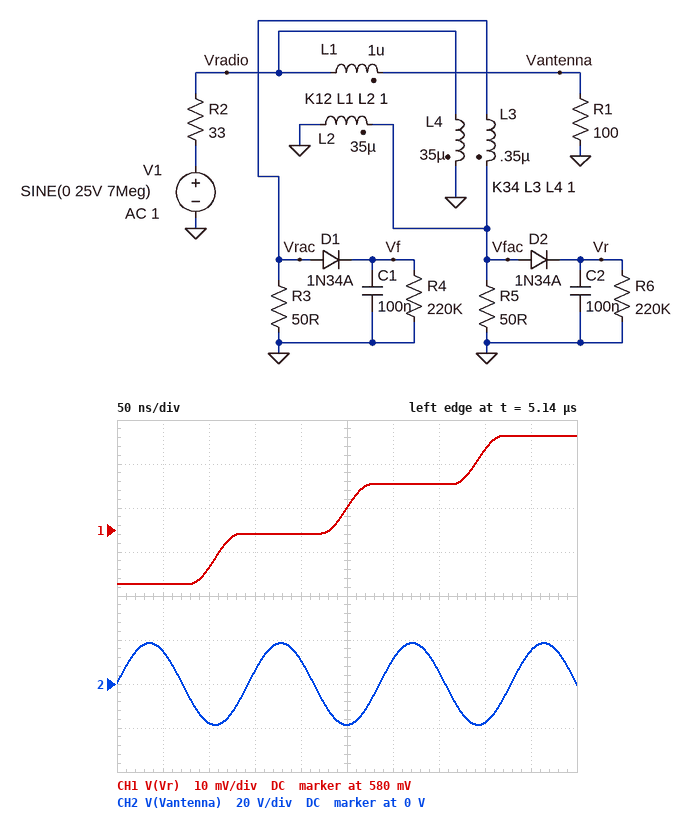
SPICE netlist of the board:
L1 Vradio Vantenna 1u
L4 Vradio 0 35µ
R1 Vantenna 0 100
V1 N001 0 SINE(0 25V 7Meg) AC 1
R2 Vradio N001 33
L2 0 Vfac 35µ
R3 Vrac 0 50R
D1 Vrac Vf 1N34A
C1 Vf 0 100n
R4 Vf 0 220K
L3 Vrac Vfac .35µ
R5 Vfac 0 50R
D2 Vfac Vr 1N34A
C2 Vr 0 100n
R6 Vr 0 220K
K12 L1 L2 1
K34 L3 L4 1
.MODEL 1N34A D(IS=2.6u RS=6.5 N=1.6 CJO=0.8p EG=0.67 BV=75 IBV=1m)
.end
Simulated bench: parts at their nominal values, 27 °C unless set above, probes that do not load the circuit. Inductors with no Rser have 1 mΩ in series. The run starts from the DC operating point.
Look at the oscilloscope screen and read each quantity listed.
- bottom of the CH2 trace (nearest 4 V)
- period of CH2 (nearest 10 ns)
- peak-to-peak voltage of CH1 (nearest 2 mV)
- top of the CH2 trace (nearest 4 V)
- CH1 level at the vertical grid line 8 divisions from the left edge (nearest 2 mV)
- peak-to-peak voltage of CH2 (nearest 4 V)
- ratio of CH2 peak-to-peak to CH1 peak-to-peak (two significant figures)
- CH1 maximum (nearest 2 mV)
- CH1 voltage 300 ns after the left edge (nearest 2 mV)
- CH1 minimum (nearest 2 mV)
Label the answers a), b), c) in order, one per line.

a) -20 V
b) 140 ns
c) 34 mV
d) 20 V
e) 598 mV
f) 36 V
g) 1100
h) 602 mV
i) 590 mV
j) 568 mV
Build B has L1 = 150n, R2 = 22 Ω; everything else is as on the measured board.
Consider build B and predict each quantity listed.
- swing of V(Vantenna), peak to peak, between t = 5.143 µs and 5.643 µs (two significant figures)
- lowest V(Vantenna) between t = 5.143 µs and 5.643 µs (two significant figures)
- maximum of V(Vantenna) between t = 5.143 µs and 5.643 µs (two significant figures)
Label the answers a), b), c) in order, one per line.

a) 41 V
b) -20 V
c) 20 V
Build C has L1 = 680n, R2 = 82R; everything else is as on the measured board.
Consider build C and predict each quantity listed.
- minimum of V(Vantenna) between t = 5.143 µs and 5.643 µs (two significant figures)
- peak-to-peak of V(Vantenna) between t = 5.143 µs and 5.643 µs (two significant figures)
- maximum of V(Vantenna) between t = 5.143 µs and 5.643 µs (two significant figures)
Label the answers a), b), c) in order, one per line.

a) -14 V
b) 27 V
c) 14 V
